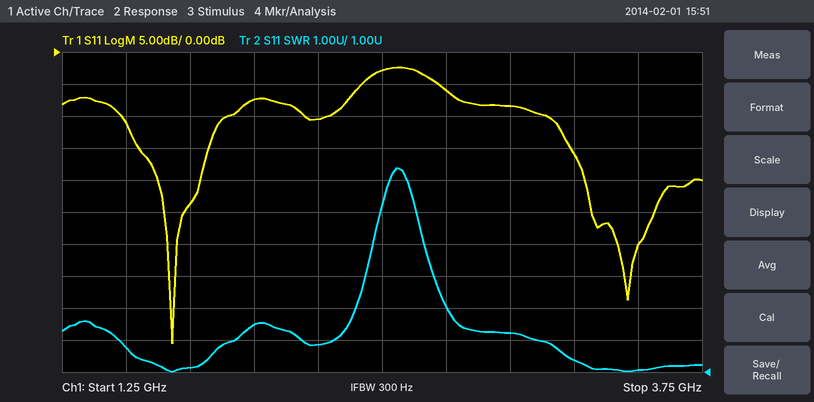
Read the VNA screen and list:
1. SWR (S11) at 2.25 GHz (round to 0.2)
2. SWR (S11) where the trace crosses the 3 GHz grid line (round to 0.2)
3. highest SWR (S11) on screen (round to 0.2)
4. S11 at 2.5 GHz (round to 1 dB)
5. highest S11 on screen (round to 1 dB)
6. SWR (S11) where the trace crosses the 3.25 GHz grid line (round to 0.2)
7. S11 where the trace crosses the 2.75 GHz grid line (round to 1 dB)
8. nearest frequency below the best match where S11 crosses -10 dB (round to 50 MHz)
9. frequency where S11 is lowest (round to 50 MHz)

1.8
2.2
7.4
-3 dB
-2 dB
1.4
-6 dB
1.50 GHz
1.70 GHz
